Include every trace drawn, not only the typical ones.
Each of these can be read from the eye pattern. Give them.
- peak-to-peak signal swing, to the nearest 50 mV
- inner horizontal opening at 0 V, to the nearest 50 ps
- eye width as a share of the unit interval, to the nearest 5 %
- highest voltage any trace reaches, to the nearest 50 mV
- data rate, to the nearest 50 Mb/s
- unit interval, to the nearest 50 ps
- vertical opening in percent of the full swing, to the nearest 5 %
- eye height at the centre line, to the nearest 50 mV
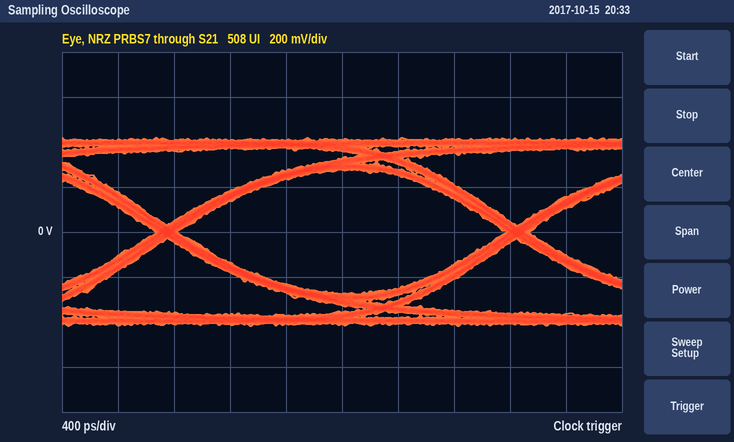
850 mV
2.35 ns
95 %
400 mV
400 Mb/s
2.50 ns
65 %
550 mV
